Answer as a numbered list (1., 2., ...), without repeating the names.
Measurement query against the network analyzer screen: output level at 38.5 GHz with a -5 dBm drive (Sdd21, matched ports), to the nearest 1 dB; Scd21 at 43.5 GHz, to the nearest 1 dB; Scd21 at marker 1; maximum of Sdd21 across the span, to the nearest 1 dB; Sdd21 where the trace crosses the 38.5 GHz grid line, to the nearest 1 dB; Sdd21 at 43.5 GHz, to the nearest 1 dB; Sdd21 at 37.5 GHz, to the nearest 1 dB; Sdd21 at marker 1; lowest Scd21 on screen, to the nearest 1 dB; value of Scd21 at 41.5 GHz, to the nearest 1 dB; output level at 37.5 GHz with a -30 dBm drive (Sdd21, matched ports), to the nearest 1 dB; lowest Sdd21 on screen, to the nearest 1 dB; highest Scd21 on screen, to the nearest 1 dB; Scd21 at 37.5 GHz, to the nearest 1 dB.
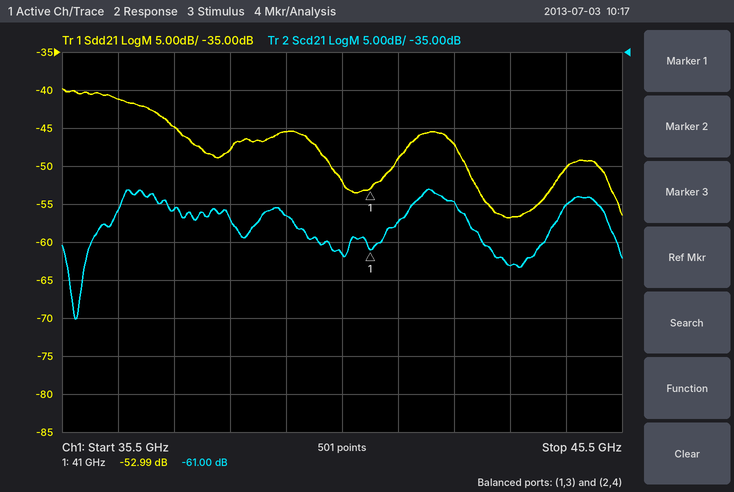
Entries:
1. -53 dBm
2. -63 dB
3. -61.00 dB
4. -40 dB
5. -48 dB
6. -57 dB
7. -45 dB
8. -52.99 dB
9. -70 dB
10. -57 dB
11. -75 dBm
12. -57 dB
13. -53 dB
14. -56 dB
